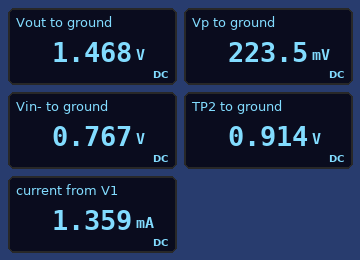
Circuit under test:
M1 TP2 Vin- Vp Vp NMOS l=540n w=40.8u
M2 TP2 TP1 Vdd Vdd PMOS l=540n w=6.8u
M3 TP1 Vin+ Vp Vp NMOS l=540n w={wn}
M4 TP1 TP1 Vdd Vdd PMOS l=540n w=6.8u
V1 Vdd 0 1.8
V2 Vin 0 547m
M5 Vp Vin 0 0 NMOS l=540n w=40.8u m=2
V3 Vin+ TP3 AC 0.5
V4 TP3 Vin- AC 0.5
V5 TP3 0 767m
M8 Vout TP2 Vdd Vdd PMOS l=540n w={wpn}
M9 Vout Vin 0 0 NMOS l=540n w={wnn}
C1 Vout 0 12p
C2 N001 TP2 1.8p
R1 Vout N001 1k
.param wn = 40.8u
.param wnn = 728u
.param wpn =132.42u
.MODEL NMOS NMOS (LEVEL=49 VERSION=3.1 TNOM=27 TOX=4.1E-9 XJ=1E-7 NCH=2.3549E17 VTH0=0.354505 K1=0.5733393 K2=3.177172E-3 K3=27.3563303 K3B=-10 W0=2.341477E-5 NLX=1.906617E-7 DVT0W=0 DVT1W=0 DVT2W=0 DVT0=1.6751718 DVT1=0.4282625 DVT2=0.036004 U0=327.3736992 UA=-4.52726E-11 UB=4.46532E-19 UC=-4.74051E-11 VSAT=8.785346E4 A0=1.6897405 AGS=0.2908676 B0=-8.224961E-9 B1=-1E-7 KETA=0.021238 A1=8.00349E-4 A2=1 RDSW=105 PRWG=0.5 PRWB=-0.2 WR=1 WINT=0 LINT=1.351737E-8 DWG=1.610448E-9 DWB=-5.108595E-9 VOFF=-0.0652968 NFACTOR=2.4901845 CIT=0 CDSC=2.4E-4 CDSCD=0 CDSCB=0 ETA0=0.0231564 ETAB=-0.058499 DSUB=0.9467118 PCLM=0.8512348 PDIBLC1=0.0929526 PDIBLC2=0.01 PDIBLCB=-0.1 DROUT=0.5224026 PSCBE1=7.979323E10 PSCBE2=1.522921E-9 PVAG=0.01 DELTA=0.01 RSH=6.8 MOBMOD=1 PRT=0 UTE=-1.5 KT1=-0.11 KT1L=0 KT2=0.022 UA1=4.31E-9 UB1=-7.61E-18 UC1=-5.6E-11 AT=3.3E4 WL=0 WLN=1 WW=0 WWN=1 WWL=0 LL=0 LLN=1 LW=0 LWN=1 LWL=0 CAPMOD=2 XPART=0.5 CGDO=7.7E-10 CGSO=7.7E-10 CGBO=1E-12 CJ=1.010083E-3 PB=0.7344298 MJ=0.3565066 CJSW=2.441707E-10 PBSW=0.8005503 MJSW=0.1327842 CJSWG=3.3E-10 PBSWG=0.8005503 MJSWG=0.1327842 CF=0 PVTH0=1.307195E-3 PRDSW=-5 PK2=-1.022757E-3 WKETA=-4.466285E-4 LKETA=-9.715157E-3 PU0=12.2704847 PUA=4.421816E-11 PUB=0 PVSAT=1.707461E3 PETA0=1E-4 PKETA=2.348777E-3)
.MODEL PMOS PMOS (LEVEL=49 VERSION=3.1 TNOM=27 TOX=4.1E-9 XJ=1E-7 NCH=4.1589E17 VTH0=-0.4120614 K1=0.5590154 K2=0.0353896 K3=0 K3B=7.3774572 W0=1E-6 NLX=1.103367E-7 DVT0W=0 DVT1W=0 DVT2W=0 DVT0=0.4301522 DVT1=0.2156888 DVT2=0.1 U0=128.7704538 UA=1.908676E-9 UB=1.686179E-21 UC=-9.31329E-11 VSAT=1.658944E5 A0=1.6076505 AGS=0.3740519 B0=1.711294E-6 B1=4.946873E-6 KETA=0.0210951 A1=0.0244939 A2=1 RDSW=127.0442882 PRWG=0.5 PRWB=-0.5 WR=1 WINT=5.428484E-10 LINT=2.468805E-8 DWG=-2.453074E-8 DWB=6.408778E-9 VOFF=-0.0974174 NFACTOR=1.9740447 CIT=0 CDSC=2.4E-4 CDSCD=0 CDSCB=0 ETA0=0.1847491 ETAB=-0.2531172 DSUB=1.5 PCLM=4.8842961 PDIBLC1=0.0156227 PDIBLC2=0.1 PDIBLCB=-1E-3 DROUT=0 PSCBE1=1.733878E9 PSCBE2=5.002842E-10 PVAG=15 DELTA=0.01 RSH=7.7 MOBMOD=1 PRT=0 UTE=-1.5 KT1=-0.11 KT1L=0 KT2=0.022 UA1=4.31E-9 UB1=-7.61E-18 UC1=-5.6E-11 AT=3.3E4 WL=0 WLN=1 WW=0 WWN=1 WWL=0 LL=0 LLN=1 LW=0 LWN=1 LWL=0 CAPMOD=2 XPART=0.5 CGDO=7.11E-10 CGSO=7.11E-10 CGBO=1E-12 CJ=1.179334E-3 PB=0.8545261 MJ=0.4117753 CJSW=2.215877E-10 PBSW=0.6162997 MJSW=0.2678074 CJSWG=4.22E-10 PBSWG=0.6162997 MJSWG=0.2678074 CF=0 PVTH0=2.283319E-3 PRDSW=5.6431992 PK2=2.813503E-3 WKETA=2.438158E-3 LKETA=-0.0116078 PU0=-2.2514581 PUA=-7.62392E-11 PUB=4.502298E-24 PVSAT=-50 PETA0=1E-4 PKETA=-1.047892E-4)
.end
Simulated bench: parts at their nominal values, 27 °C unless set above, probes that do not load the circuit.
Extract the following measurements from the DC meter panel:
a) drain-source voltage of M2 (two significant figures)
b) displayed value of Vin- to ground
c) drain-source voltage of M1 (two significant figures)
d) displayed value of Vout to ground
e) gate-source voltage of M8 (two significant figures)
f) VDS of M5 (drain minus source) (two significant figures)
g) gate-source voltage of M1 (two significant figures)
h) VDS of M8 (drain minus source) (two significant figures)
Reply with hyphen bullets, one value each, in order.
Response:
- -890 mV
- 0.767 V
- 690 mV
- 1.468 V
- -890 mV
- 220 mV
- 540 mV
- -330 mV
